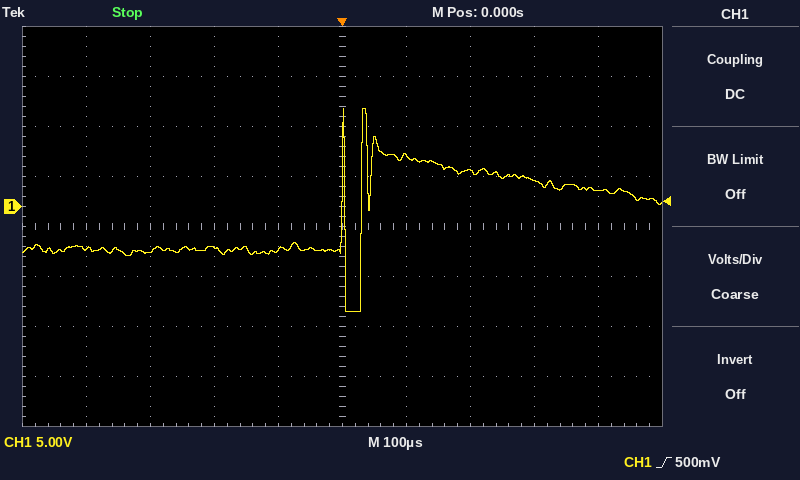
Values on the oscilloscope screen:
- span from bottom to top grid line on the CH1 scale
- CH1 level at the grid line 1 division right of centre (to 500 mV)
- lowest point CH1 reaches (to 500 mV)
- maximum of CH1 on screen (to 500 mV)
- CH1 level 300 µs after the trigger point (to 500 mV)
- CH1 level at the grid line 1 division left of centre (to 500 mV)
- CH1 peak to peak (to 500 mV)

40 V
5.0 V
-10.5 V
10.0 V
2.5 V
-4.5 V
20.5 V
